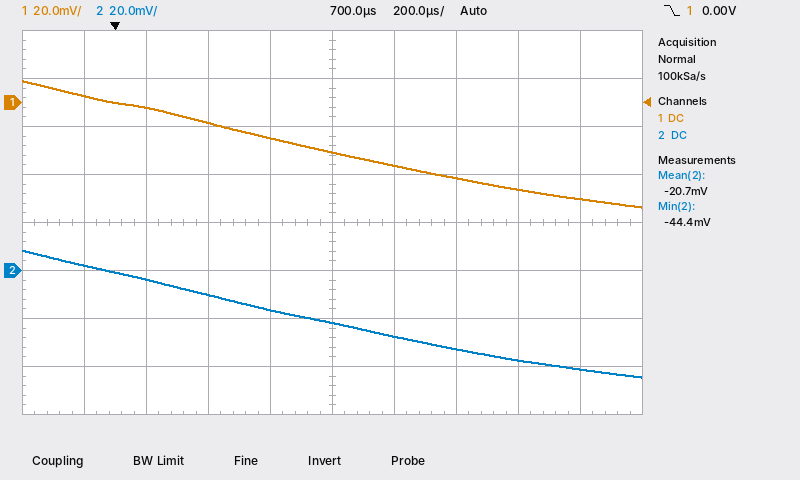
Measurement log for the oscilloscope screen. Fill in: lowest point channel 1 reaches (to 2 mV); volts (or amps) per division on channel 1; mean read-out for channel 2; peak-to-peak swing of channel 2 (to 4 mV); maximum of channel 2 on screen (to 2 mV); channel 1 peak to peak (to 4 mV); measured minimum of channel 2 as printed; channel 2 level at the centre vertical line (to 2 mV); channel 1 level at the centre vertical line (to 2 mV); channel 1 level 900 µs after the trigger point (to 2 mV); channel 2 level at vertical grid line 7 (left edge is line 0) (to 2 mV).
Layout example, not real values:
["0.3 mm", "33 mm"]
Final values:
["-44 mV", "20 mV", "-20.7 mV", "52 mV", "8 mV", "52 mV", "-44.4 mV", "-22 mV", "-20 mV", "-26 mV", "-32 mV"]
